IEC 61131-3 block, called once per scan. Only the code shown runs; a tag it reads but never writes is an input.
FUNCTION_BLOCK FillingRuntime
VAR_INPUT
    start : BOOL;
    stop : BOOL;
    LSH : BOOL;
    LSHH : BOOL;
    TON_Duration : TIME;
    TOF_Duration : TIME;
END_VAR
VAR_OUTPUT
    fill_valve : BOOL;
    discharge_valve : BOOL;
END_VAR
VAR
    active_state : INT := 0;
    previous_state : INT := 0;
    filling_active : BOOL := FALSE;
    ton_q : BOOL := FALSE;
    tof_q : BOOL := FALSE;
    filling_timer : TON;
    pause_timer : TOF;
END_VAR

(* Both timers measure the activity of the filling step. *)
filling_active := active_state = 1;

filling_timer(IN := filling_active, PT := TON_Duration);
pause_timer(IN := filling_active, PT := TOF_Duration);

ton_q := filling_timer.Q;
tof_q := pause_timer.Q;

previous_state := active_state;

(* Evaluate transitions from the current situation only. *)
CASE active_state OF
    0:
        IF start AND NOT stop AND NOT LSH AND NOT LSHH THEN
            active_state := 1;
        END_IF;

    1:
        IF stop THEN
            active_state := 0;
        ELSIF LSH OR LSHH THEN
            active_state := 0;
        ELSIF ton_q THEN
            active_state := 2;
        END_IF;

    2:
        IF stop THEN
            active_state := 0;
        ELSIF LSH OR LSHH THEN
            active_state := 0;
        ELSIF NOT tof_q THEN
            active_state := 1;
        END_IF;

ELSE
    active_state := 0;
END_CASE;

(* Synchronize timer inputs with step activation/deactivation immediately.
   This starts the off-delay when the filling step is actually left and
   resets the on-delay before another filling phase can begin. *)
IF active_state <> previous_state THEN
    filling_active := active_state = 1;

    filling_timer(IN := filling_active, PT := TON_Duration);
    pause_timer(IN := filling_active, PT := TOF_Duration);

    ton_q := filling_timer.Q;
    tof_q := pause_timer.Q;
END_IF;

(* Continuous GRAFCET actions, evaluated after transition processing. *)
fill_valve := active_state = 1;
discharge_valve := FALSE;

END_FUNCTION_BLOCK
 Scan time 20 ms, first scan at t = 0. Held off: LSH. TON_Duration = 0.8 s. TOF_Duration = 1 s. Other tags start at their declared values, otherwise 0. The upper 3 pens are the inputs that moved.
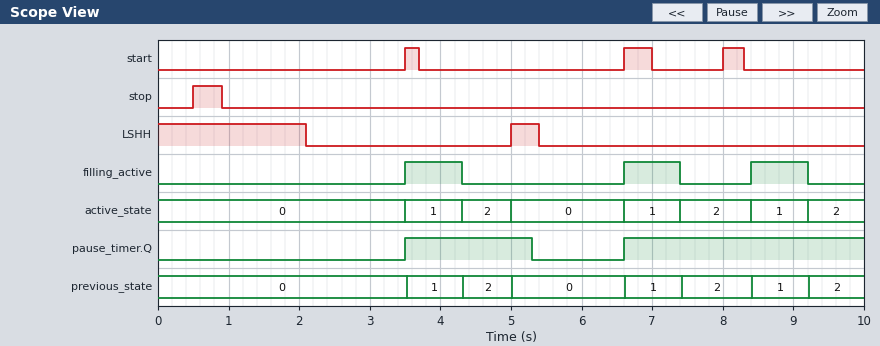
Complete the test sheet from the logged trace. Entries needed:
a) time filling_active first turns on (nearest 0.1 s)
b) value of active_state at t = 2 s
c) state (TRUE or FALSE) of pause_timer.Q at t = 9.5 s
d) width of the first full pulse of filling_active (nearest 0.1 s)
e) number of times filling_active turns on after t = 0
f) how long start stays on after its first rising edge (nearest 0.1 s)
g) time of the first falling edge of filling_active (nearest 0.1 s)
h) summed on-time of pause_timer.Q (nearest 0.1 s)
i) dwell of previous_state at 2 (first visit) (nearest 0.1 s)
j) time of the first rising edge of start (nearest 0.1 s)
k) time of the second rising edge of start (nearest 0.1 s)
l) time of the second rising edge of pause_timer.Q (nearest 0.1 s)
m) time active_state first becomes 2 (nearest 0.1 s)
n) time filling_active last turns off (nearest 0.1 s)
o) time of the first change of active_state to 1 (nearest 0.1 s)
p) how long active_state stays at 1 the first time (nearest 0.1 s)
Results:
3.5 s
0
TRUE
0.8 s
3
0.2 s
4.3 s
5.2 s
0.7 s
3.5 s
6.6 s
6.6 s
4.3 s
9.2 s
3.5 s
0.8 s
